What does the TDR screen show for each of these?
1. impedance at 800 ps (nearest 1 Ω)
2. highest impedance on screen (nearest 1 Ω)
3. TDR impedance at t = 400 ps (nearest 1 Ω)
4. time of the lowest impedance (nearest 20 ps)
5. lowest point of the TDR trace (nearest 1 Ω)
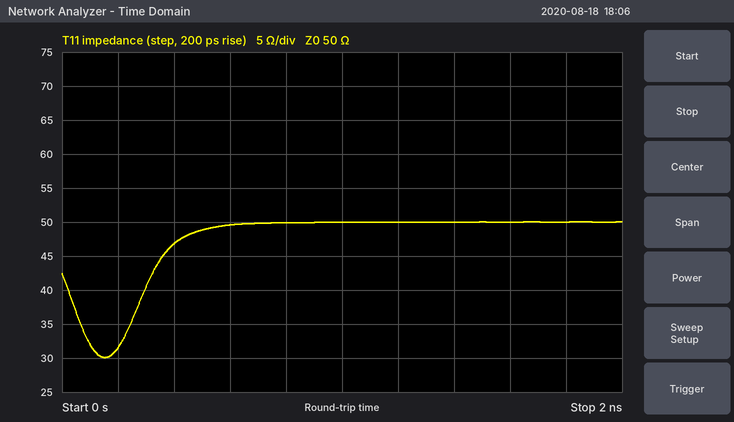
50 Ω
50 Ω
47 Ω
160 ps
30 Ω
